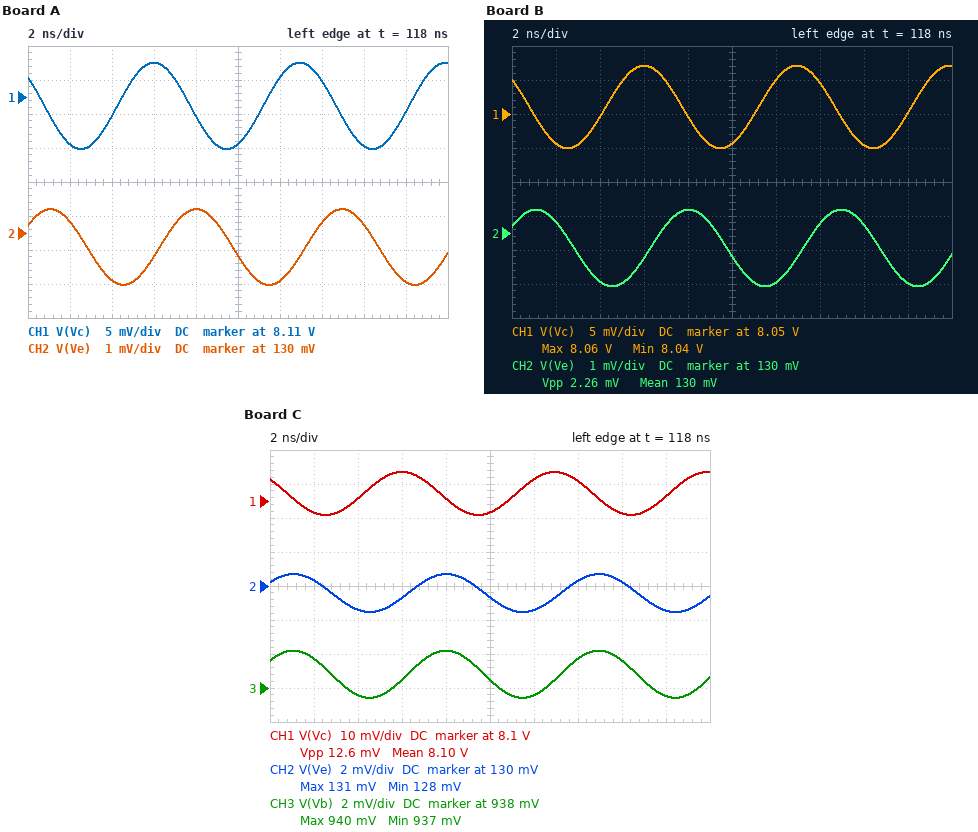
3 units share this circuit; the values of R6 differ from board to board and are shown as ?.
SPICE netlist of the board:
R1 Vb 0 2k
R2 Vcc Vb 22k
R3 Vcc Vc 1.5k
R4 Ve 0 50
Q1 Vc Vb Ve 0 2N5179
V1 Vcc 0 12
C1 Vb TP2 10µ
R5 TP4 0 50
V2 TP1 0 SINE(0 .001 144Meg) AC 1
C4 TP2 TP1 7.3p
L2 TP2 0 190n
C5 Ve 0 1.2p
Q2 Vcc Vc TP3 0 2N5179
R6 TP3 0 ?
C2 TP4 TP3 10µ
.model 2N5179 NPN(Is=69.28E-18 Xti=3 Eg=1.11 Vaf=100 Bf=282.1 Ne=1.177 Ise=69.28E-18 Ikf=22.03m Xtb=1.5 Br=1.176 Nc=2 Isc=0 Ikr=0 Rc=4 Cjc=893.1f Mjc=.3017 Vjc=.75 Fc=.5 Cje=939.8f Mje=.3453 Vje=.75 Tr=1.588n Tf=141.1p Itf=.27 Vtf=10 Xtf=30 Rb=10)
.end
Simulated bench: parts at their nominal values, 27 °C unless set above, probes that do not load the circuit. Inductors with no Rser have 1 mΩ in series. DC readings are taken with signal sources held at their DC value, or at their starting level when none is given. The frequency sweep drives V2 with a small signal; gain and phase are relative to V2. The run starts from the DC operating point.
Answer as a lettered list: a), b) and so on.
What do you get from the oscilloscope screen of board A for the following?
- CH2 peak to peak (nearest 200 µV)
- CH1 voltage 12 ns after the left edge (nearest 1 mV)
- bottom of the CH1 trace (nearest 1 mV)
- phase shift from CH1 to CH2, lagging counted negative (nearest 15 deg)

a) 2.2 mV
b) 8.113 V
c) 8.102 V
d) -105 deg
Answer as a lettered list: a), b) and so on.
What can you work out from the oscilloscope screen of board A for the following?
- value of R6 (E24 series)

a) 2.7 kΩ
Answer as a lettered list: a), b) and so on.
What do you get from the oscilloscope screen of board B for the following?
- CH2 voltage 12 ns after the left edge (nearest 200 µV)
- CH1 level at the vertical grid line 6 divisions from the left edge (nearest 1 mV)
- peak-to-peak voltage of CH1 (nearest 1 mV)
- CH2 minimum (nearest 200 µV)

a) 128.6 mV
b) 8.055 V
c) 12 mV
d) 128.4 mV
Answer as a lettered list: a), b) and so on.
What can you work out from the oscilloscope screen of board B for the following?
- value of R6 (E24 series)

a) 1.3 kΩ
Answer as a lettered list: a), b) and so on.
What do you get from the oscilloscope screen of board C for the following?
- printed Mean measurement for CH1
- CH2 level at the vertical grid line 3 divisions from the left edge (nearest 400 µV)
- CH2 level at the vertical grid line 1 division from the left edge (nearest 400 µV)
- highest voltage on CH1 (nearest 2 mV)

a) 8.10 V
b) 129.2 mV
c) 130.4 mV
d) 8.108 V
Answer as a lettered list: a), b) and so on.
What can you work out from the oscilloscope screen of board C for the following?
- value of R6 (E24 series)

a) 2.4 kΩ
